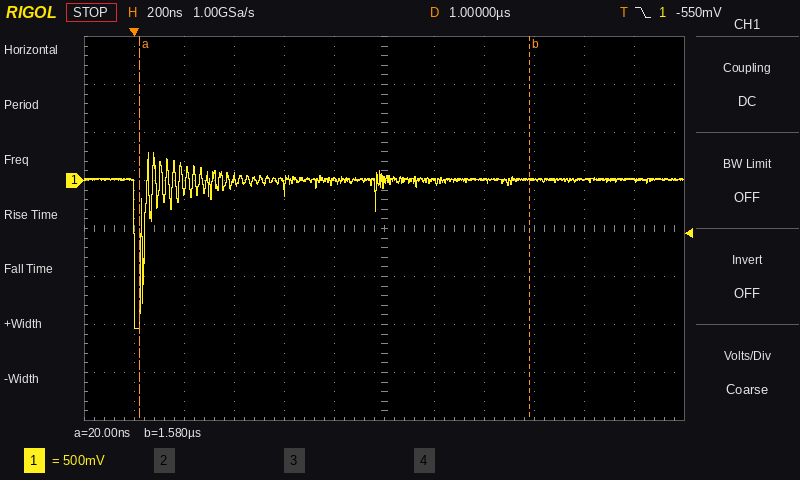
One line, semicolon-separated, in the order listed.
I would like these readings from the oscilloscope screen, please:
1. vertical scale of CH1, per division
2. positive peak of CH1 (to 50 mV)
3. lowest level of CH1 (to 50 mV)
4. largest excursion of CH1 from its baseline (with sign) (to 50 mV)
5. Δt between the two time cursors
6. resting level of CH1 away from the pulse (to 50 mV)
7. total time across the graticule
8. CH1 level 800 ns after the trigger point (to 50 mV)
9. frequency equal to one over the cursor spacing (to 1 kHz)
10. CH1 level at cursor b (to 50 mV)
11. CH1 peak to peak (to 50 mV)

500 mV; 300 mV; -1.55 V; -1.55 V; 1.56 µs; 0 mV; 2.4 µs; 0 mV; 641 kHz; 0 mV; 1.85 V
